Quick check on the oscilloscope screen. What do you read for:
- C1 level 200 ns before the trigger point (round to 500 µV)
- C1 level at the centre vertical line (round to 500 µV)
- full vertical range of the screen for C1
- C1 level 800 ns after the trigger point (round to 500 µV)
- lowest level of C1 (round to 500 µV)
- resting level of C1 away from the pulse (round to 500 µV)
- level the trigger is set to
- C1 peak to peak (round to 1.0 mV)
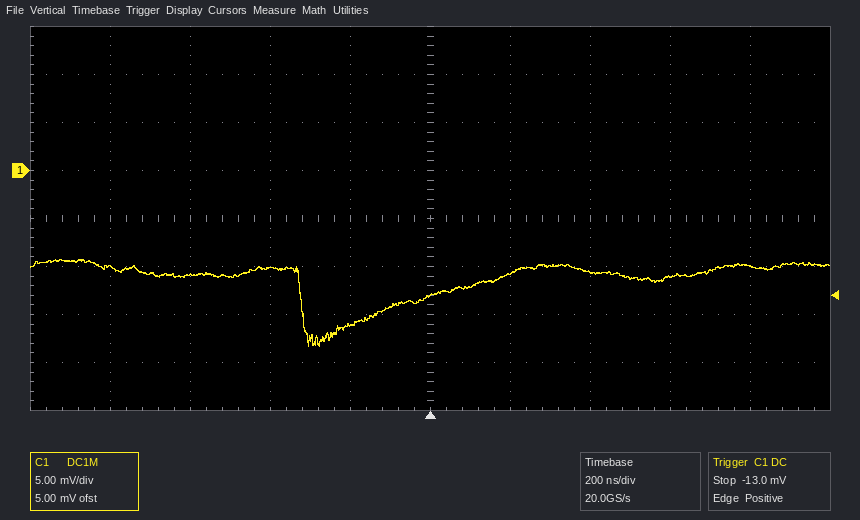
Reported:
-16.0 mV
-13.0 mV
40 mV
-10.0 mV
-18.5 mV
-10.5 mV
-13.0 mV
9.0 mV
